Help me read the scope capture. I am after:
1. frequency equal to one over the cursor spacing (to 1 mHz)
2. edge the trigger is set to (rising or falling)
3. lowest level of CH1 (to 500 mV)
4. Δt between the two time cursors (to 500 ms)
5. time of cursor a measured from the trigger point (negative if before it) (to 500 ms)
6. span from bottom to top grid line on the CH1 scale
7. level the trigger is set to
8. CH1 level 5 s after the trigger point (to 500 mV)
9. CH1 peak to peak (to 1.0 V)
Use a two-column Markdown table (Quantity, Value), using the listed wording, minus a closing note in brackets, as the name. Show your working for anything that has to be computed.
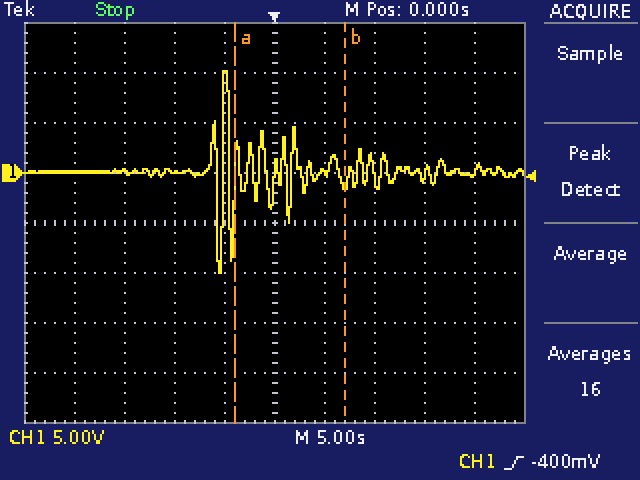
| Quantity | Value |
|---|---|
| frequency equal to one over the cursor spacing | 1 / 11.0 s ≈ 91 mHz |
| edge the trigger is set to | rising |
| lowest level of CH1 | -10.0 V |
| Δt between the two time cursors | 11.0 s |
| time of cursor a measured from the trigger point (negative if before it) | -4.0 s |
| span from bottom to top grid line on the CH1 scale | 40 V |
| level the trigger is set to | -400 mV |
| CH1 level 5 s after the trigger point | 0.0 V |
| CH1 peak to peak | 20.0 V |
